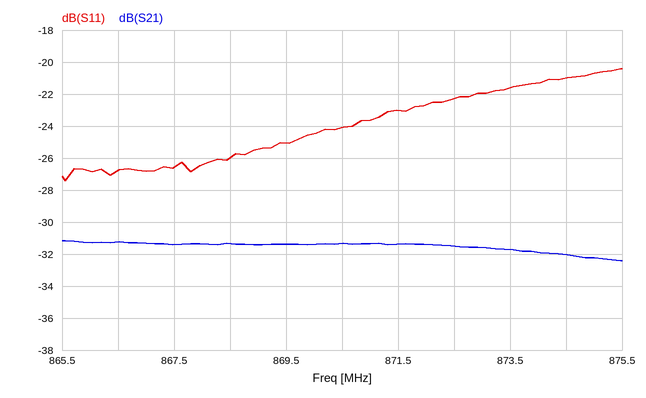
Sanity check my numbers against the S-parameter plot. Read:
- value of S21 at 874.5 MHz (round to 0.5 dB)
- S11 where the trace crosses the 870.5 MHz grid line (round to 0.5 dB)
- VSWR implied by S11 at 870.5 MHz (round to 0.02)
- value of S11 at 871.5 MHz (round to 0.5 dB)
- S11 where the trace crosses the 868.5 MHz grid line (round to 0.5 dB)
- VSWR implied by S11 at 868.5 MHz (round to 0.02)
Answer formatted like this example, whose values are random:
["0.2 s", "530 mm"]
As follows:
["-32.0 dB", "-24.0 dB", "1.14", "-23.0 dB", "-26.0 dB", "1.10"]
